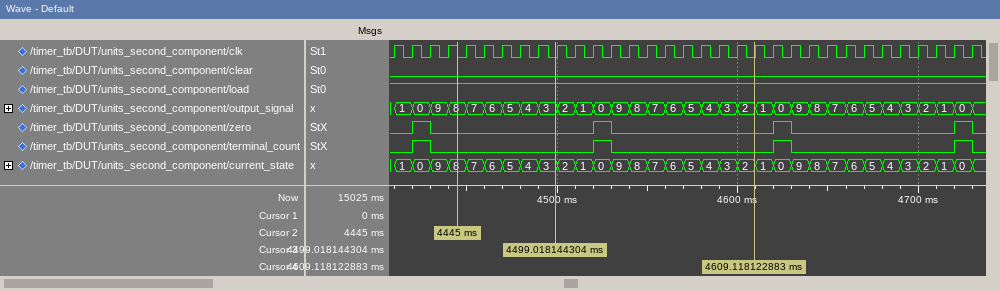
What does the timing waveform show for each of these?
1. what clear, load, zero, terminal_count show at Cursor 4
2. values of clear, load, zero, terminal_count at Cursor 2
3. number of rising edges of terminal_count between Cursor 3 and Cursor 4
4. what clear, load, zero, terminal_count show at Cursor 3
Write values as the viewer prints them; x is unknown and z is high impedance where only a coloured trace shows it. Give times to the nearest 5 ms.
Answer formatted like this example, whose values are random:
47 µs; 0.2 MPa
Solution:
clear=0, load=1, zero=0, terminal_count=0; clear=0, load=1, zero=0, terminal_count=0; 1; clear=0, load=1, zero=0, terminal_count=0
